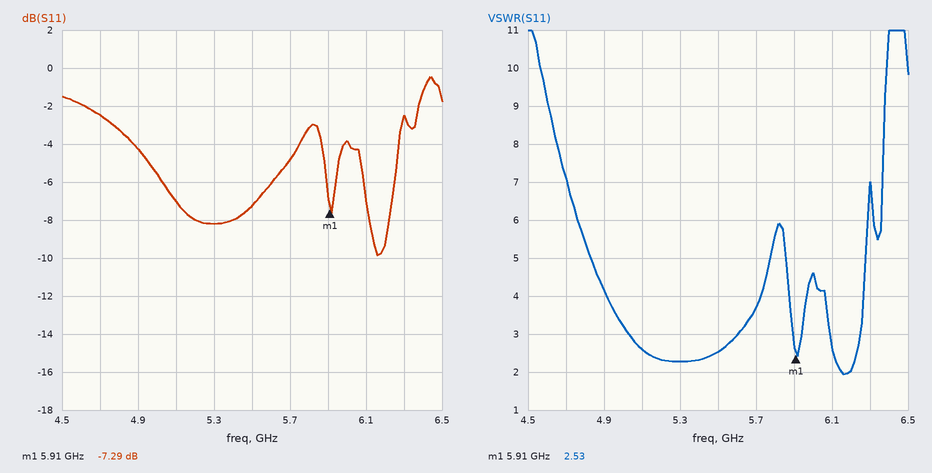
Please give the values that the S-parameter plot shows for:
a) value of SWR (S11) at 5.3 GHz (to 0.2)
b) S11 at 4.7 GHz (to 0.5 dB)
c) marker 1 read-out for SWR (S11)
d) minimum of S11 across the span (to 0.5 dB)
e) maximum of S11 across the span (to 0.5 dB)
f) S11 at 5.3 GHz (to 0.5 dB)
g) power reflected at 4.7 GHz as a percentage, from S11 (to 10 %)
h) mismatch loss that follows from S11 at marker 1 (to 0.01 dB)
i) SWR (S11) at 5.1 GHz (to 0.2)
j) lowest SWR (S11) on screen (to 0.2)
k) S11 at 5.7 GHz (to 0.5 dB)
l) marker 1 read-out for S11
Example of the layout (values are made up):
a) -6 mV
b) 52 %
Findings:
a) 2.2
b) -2.5 dB
c) 2.53
d) -10.0 dB
e) -0.5 dB
f) -8.0 dB
g) 60 %
h) 0.90 dB
i) 2.6
j) 2.0
k) -5.0 dB
l) -7.29 dB
